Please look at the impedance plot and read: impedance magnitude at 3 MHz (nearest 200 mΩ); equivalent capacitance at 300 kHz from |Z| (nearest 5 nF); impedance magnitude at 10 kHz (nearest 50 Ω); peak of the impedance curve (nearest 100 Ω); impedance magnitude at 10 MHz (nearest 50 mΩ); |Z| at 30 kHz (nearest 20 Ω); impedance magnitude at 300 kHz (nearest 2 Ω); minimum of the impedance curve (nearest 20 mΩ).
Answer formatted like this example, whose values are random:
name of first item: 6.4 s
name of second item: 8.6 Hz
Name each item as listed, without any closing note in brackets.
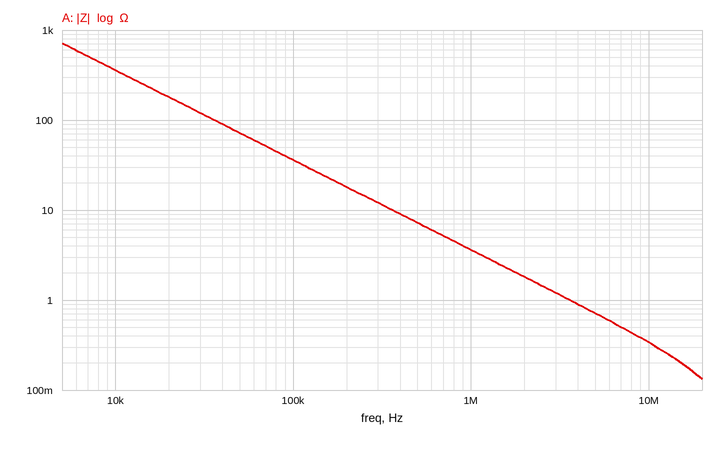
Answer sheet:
impedance magnitude at 3 MHz: 1.2 Ω
equivalent capacitance at 300 kHz from |Z|: 45 nF
impedance magnitude at 10 kHz: 350 Ω
peak of the impedance curve: 700 Ω
impedance magnitude at 10 MHz: 350 mΩ
|Z| at 30 kHz: 120 Ω
impedance magnitude at 300 kHz: 12 Ω
minimum of the impedance curve: 140 mΩ
